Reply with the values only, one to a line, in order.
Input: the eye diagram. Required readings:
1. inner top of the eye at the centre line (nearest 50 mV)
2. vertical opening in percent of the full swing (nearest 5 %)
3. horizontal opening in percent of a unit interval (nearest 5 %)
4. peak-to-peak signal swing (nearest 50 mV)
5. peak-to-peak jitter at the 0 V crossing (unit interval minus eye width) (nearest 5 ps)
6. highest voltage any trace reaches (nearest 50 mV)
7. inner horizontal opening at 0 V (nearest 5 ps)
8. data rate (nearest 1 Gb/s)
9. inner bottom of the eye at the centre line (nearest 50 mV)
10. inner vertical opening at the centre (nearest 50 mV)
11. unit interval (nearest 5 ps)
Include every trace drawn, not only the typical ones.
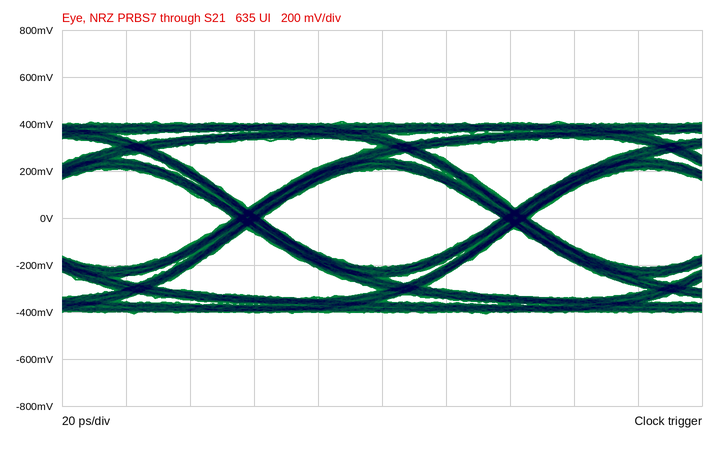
200 mV
50 %
90 %
800 mV
10 ps
400 mV
75 ps
12 Gb/s
-200 mV
400 mV
85 ps
